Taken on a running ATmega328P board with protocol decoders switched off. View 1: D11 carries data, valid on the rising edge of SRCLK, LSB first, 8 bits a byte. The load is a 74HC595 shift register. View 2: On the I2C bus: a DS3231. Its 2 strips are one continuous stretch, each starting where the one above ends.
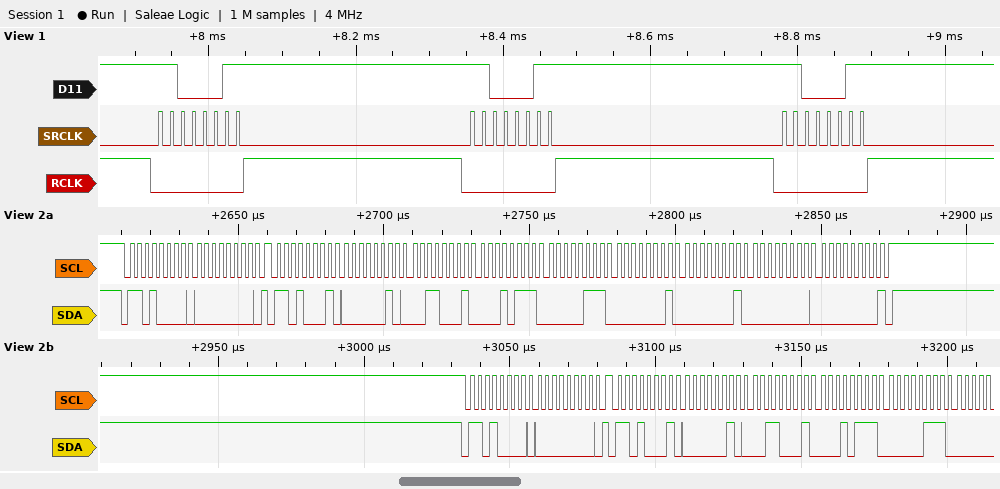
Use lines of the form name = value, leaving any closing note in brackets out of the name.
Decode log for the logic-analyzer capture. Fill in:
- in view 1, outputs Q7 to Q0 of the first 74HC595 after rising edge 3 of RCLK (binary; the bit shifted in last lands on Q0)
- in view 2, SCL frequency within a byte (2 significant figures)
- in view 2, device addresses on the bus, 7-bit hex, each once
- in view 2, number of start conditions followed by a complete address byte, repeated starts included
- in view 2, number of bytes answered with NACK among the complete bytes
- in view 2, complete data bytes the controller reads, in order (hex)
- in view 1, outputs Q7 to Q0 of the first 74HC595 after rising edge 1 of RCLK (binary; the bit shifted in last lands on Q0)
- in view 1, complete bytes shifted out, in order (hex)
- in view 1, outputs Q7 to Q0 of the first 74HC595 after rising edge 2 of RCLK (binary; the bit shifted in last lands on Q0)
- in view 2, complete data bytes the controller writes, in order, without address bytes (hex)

in view 1, outputs Q7 to Q0 of the first 74HC595 after rising edge 3 of RCLK = 11000011
in view 2, SCL frequency within a byte = 400 kHz
in view 2, device addresses on the bus, 7-bit hex, each once = 0x68
in view 2, number of start conditions followed by a complete address byte, repeated starts included = 4
in view 2, number of bytes answered with NACK among the complete bytes = 1
in view 2, complete data bytes the controller reads, in order = 02 31 17 07 01 01 00 00 02 31 17 07
in view 1, outputs Q7 to Q0 of the first 74HC595 after rising edge 1 of RCLK = 11000011
in view 1, complete bytes shifted out, in order = 0xC3 0xC3 0xC3
in view 1, outputs Q7 to Q0 of the first 74HC595 after rising edge 2 of RCLK = 11000011
in view 2, complete data bytes the controller writes, in order, without address bytes = 00 00
